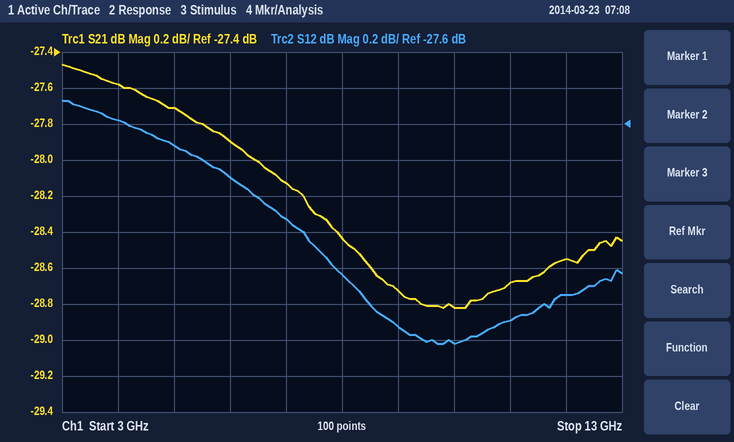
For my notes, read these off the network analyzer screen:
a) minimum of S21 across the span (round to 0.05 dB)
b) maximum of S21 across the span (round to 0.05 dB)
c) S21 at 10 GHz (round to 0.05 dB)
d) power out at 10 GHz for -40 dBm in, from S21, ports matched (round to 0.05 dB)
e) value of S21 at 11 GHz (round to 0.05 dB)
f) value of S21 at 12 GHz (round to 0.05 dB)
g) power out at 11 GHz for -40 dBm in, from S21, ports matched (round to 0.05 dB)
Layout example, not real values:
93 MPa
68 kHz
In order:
-28.80 dB
-27.45 dB
-28.80 dB
-68.80 dBm
-28.70 dB
-28.55 dB
-68.70 dBm
